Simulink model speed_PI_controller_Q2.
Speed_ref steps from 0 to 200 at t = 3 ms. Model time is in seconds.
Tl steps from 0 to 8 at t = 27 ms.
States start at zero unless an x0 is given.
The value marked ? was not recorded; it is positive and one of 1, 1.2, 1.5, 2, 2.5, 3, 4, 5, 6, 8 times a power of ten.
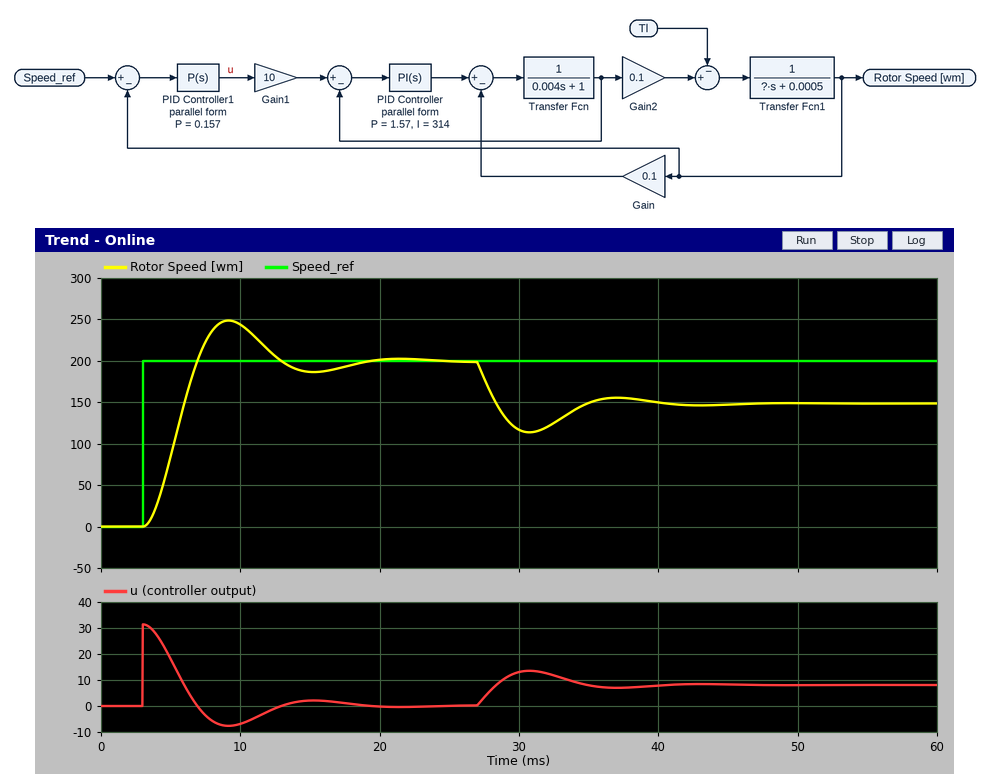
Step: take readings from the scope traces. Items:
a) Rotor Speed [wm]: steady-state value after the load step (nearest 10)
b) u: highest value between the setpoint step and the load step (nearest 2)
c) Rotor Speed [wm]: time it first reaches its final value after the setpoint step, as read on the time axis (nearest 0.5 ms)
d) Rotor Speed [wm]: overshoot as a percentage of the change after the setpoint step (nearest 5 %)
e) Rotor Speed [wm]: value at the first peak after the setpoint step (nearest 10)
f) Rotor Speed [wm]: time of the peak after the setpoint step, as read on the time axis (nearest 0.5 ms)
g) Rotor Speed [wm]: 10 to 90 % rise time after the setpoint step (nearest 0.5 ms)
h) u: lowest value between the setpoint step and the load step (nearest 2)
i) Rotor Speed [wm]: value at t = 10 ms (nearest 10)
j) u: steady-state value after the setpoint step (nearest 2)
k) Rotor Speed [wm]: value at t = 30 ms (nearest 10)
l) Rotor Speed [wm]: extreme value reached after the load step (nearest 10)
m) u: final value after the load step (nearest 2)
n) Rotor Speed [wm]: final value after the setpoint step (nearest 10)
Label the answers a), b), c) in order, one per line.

a) 150
b) 32
c) 7.0 ms
d) 25 %
e) 250
f) 9.0 ms
g) 2.5 ms
h) -8
i) 240
j) 0
k) 120
l) 110
m) 8
n) 200
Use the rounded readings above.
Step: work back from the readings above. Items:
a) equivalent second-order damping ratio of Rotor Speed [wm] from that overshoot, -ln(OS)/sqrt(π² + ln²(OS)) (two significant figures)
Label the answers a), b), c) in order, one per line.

a) 0.40
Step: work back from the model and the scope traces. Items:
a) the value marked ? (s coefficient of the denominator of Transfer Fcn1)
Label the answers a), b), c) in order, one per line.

a) 0.0002
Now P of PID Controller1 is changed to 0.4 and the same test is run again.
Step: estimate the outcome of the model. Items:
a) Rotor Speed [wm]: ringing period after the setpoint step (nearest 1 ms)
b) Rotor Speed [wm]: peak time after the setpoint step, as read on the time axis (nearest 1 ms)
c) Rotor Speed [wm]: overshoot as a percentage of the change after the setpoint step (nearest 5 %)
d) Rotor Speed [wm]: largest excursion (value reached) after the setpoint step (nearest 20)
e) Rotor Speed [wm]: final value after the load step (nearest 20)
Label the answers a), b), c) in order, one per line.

a) 7 ms
b) 7 ms
c) 45 %
d) 280
e) 180
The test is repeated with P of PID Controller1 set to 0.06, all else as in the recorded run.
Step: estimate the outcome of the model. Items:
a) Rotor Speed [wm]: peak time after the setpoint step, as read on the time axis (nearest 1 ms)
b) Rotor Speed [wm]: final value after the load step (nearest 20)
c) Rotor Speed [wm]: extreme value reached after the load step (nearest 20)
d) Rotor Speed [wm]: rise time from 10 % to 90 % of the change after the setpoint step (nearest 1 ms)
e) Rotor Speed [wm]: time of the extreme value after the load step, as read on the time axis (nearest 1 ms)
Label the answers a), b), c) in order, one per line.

a) 15 ms
b) 60
c) 40
d) 6 ms
e) 35 ms
